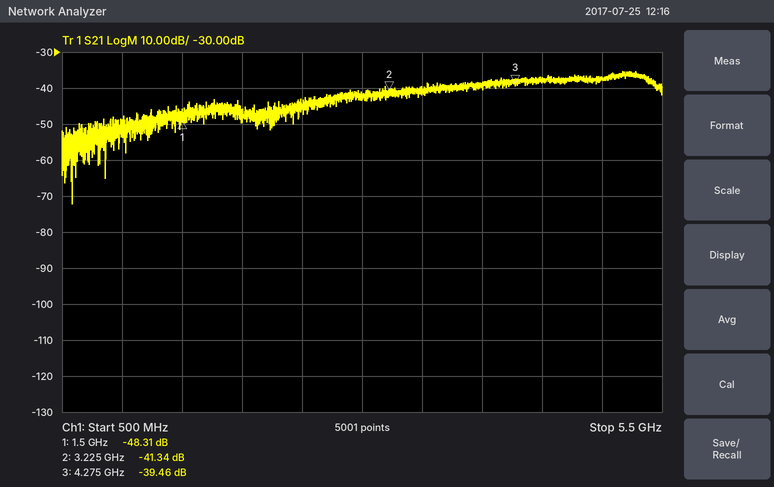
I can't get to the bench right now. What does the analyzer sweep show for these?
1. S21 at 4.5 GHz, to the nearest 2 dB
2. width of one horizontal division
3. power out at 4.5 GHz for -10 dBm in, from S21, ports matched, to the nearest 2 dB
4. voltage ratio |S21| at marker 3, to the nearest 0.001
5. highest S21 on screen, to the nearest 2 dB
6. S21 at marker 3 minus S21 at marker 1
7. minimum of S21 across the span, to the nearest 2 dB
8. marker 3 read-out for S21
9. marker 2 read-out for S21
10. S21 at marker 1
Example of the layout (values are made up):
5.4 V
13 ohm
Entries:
-38 dB
500 MHz
-48 dBm
0.011
-36 dB
8.85 dB
-72 dB
-39.46 dB
-41.34 dB
-48.31 dB
